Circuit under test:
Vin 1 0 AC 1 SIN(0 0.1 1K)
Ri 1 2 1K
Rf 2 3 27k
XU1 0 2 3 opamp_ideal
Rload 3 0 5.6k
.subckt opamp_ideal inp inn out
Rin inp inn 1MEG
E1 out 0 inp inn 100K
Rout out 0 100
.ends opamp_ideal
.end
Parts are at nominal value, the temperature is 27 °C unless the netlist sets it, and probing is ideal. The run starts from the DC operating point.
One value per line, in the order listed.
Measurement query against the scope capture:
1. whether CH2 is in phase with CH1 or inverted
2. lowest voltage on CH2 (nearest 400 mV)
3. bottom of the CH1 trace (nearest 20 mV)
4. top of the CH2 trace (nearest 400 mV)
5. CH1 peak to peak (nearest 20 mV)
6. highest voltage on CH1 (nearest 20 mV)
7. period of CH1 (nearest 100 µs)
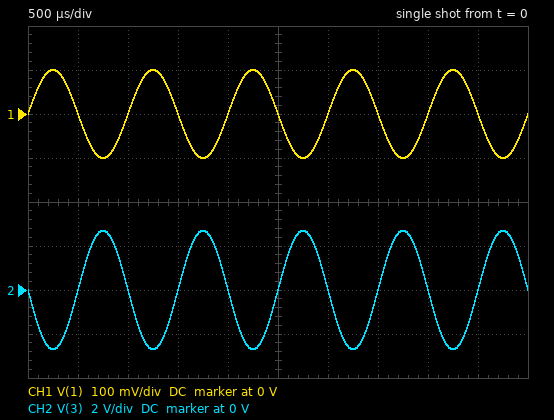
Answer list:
inverted
-2.8 V
-100 mV
2.8 V
200 mV
100 mV
1.0 ms
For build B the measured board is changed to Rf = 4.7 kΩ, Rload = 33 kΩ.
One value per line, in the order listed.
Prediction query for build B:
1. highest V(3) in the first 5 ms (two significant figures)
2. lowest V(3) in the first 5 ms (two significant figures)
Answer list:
470 mV
-470 mV
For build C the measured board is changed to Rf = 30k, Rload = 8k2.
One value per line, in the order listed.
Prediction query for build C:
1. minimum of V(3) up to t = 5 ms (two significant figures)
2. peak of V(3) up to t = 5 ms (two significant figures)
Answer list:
-3.0 V
3.0 V
